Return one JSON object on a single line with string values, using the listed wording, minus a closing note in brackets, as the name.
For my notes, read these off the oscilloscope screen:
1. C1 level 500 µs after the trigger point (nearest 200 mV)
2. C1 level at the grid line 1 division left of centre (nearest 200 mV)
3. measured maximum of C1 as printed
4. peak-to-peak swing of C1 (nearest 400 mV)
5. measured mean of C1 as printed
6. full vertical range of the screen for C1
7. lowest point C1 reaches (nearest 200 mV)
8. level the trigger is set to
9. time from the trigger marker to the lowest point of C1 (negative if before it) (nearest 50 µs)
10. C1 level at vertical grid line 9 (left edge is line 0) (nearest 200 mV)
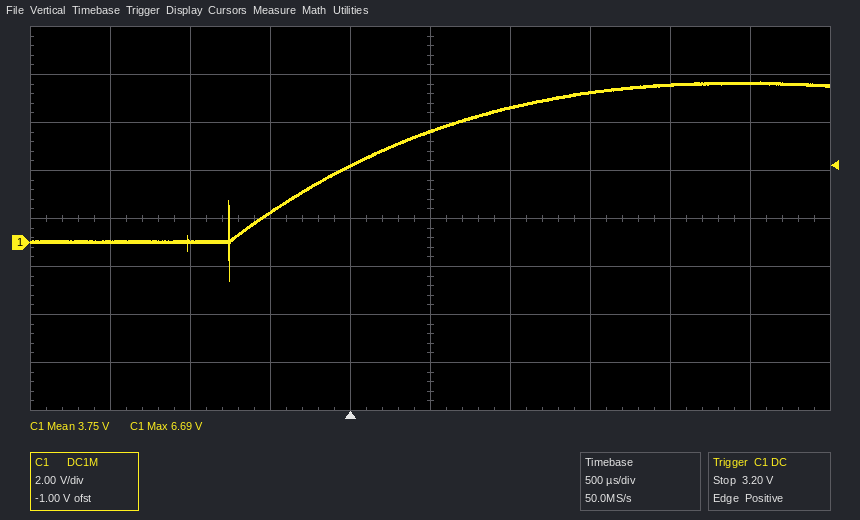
{"C1 level 500 µs after the trigger point": "4.6 V", "C1 level at the grid line 1 division left of centre": "3.2 V", "measured maximum of C1 as printed": "6.69 V", "peak-to-peak swing of C1": "8.4 V", "measured mean of C1 as printed": "3.75 V", "full vertical range of the screen for C1": "16 V", "lowest point C1 reaches": "-1.6 V", "level the trigger is set to": "3.20 V", "time from the trigger marker to the lowest point of C1 (negative if before it)": "-750 µs", "C1 level at vertical grid line 9 (left edge is line 0)": "6.6 V"}
